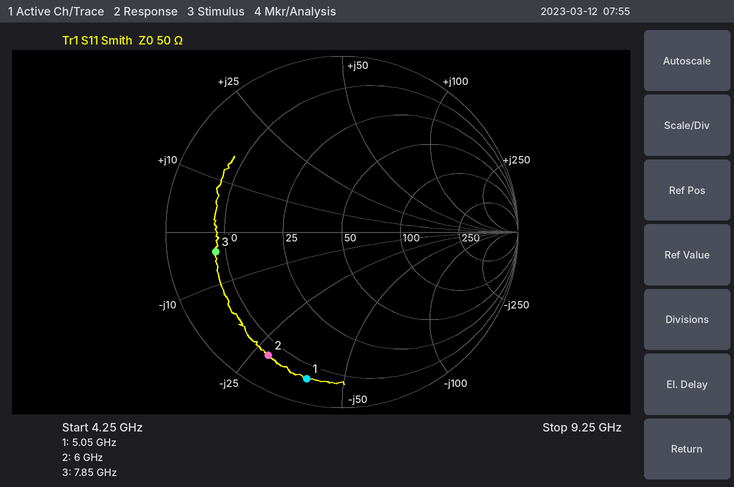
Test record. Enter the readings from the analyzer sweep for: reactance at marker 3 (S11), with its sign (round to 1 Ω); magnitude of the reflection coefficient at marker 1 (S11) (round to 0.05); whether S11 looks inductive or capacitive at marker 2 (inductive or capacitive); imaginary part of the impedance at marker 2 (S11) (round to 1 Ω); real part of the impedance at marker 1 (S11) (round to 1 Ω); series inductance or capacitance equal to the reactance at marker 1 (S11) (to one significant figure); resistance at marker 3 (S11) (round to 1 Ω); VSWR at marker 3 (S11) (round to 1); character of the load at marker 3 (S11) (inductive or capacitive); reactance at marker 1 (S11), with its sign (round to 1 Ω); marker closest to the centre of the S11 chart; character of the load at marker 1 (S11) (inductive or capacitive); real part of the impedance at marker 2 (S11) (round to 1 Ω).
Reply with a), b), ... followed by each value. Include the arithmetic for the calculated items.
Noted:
a) -4 Ω
b) 0.85
c) capacitive
d) -28 Ω
e) 6 Ω
f) C = 1/(2π × 5.05 GHz × 39 Ω) ≈ 808 fF, so 800 fF to one significant figure
g) 8 Ω
h) 6
i) capacitive
j) -39 Ω
k) marker 3
l) capacitive
m) 7 Ω
